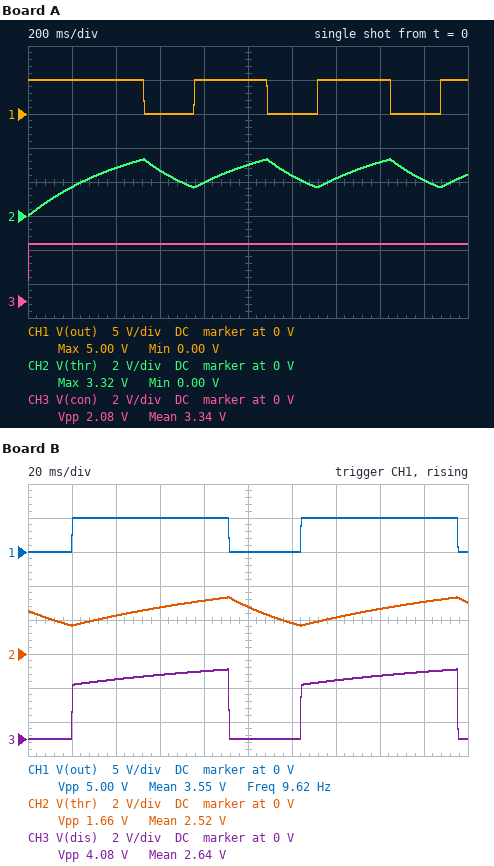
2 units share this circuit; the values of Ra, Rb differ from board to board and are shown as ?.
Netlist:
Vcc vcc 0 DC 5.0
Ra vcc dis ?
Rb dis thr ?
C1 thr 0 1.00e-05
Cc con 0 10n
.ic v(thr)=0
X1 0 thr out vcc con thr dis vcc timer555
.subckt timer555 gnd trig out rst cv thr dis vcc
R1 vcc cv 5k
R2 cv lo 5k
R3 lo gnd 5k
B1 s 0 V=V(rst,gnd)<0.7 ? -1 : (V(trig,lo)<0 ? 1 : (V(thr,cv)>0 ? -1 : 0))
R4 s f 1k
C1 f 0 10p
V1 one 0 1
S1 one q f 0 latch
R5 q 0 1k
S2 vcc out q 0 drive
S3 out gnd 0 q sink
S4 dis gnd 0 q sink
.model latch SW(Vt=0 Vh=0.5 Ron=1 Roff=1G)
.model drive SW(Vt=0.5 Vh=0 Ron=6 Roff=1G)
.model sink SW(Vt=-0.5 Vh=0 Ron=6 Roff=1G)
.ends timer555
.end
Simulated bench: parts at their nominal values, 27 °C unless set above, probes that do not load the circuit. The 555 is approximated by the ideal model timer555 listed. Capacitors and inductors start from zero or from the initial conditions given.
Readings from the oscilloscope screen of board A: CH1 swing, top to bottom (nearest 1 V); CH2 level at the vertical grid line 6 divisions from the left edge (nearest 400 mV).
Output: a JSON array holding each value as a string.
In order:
["5 V", "2.4 V"]
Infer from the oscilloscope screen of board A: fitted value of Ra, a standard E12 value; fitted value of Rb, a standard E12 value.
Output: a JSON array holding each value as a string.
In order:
["15 kΩ", "33 kΩ"]
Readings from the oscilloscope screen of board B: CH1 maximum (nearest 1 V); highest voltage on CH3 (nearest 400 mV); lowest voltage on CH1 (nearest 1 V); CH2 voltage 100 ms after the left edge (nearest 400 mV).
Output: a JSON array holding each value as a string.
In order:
["5 V", "4.0 V", "0 V", "2.8 V"]
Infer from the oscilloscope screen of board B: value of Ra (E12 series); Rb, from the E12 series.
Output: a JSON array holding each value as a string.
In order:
["5.6 kΩ", "4.7 kΩ"]
